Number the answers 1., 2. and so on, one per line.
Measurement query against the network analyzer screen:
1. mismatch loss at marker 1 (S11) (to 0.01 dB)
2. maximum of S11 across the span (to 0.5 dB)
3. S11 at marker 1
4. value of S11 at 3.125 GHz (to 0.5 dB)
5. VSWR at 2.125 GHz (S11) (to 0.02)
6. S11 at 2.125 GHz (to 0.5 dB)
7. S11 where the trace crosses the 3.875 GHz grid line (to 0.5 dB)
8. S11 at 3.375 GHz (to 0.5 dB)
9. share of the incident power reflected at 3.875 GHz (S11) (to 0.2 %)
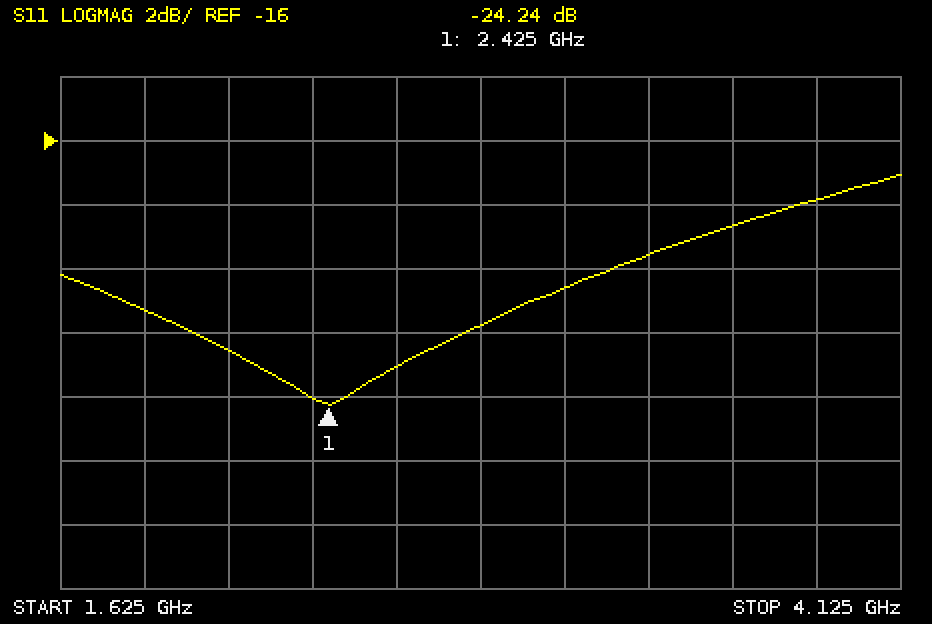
1. 0.02 dB
2. -17.0 dB
3. -24.24 dB
4. -20.5 dB
5. 1.16
6. -22.5 dB
7. -18.0 dB
8. -19.5 dB
9. 1.6 %
